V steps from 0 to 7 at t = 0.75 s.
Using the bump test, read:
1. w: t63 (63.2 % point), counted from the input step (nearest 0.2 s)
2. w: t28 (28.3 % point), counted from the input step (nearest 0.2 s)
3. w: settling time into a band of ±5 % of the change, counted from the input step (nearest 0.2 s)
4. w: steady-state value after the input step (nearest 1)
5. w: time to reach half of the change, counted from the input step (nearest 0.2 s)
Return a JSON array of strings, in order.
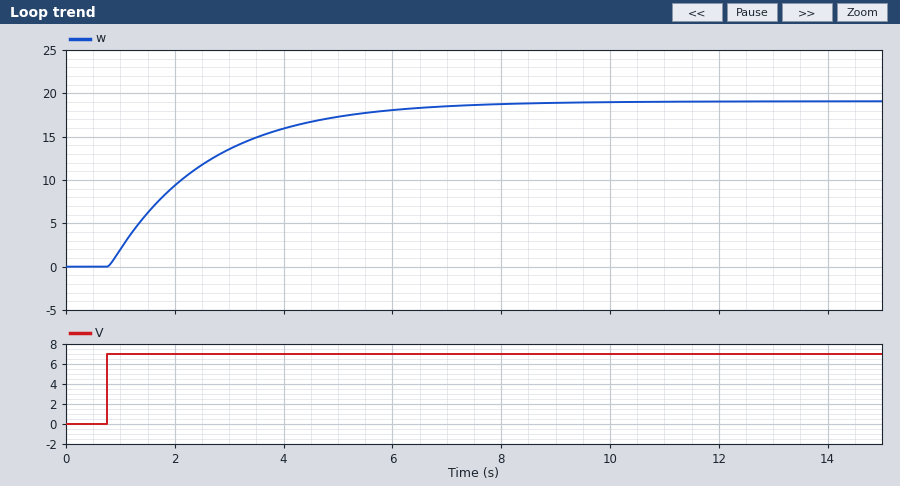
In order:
["1.8 s", "0.6 s", "5.4 s", "19", "1.2 s"]
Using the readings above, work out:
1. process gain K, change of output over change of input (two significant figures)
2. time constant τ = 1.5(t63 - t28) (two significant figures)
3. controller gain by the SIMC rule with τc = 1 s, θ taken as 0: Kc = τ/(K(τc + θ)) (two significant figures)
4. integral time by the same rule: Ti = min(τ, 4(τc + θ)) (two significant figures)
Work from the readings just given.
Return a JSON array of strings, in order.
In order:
["2.7", "1.8 s", "0.67", "1.8 s"]
